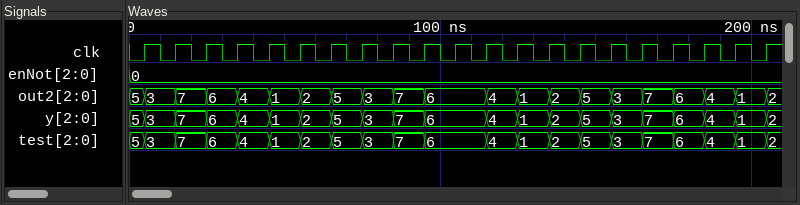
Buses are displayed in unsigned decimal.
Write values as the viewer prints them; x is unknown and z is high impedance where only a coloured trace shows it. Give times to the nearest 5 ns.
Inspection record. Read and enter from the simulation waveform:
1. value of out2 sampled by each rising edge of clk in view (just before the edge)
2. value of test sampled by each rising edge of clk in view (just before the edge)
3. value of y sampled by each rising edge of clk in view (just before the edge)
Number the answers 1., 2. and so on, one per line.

1. 5, 3, 7, 6, 4, 1, 2, 5, 3, 7, 6, 6, 4, 1, 2, 5, 3, 7, 6, 4, 1
2. 5, 3, 7, 6, 4, 1, 2, 5, 3, 7, 6, 6, 4, 1, 2, 5, 3, 7, 6, 4, 1
3. 5, 3, 7, 6, 4, 1, 2, 5, 3, 7, 6, 6, 4, 1, 2, 5, 3, 7, 6, 4, 1
